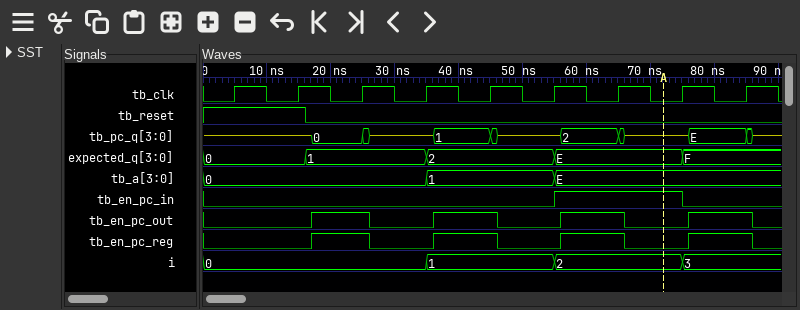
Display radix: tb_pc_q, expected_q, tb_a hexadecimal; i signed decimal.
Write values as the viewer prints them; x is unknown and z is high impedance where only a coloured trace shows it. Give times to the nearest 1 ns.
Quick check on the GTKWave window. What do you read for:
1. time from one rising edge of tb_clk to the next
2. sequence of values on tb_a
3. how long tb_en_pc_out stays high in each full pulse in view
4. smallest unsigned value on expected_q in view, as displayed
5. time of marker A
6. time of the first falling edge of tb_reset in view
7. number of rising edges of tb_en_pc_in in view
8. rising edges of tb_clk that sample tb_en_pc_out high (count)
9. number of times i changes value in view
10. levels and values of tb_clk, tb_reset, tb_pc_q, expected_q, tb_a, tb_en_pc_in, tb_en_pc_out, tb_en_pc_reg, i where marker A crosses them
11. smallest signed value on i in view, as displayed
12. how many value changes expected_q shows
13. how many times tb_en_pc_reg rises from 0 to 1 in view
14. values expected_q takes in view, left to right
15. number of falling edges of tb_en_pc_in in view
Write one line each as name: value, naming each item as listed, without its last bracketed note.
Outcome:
time from one rising edge of tb_clk to the next: 10 ns
sequence of values on tb_a: 0, 1, E
how long tb_en_pc_out stays high in each full pulse in view: 9 ns, 10 ns, 10 ns, 10 ns
smallest unsigned value on expected_q in view, as displayed: 0
time of marker A: 72 ns
time of the first falling edge of tb_reset in view: 16 ns
number of rising edges of tb_en_pc_in in view: 1
rising edges of tb_clk that sample tb_en_pc_out high: 4
number of times i changes value in view: 3
levels and values of tb_clk, tb_reset, tb_pc_q, expected_q, tb_a, tb_en_pc_in, tb_en_pc_out, tb_en_pc_reg, i where marker A crosses them: tb_clk=0, tb_reset=0, tb_pc_q=z, expected_q=E, tb_a=E, tb_en_pc_in=1, tb_en_pc_out=0, tb_en_pc_reg=0, i=2
smallest signed value on i in view, as displayed: 0
how many value changes expected_q shows: 4
how many times tb_en_pc_reg rises from 0 to 1 in view: 4
values expected_q takes in view, left to right: 0, 1, 2, E, F
number of falling edges of tb_en_pc_in in view: 1
